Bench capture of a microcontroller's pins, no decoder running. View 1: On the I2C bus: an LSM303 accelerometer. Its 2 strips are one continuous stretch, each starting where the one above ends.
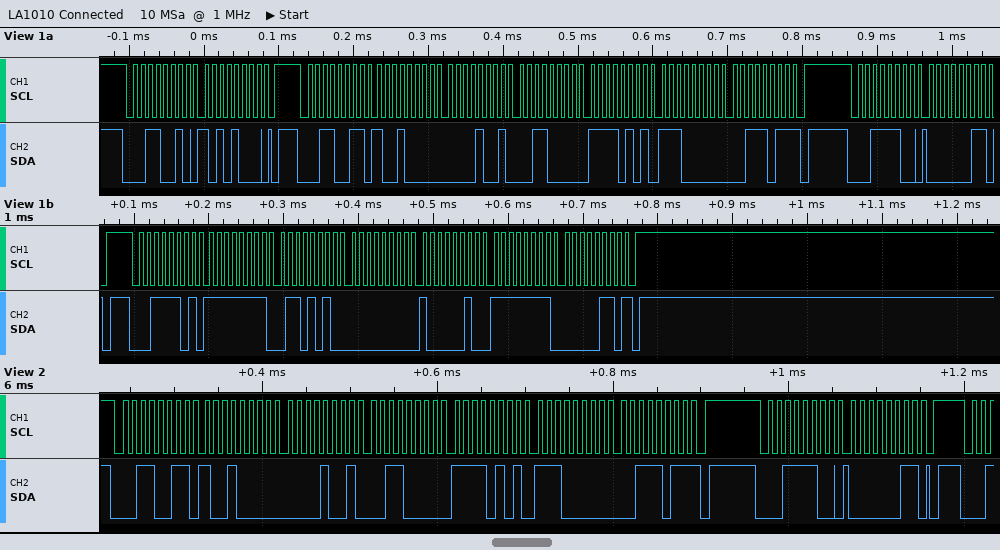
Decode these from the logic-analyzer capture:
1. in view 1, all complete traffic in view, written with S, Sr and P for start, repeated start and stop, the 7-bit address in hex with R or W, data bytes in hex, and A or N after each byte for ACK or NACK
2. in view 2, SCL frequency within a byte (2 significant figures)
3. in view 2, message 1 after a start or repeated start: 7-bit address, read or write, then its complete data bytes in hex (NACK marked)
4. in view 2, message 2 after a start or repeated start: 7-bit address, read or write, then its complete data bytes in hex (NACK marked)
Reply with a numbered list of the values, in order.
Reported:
1. S 19W A A8 A P S 19R A 90 A 09 A 30 A F5 A E0 A 3B N P S 1EW A 03 A P S 1ER A FF A 6A A 00 A 82 A FF A 06 N P
2. 100 kHz
3. 0x19 read: 90 09 30 F5 E0 3B NACK
4. 0x1E write: 03
